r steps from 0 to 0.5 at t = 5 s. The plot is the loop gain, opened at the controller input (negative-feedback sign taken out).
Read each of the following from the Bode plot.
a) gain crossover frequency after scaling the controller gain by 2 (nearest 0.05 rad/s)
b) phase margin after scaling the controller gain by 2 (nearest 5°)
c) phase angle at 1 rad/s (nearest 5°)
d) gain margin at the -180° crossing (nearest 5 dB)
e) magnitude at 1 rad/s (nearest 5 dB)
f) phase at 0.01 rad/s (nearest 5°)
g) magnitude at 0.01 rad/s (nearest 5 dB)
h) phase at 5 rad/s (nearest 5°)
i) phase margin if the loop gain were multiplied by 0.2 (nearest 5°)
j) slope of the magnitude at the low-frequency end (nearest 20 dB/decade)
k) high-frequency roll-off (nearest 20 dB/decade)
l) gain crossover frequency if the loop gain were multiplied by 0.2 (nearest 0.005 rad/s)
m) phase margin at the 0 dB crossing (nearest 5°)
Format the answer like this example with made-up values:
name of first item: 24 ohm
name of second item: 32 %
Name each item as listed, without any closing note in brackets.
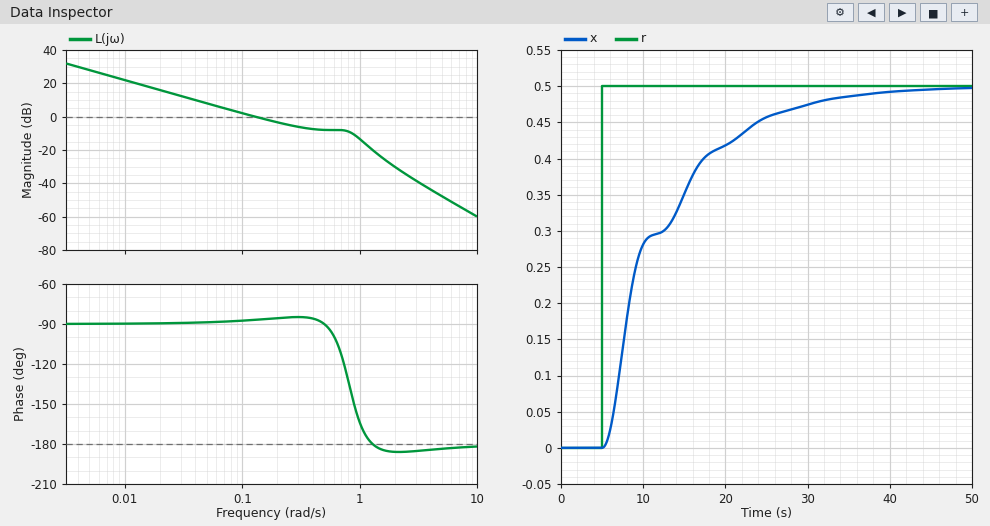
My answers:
gain crossover frequency after scaling the controller gain by 2: 0.30 rad/s
phase margin after scaling the controller gain by 2: 95°
phase angle at 1 rad/s: -165°
gain margin at the -180° crossing: 20 dB
magnitude at 1 rad/s: -15 dB
phase at 0.01 rad/s: -90°
magnitude at 0.01 rad/s: 20 dB
phase at 5 rad/s: -185°
phase margin if the loop gain were multiplied by 0.2: 90°
slope of the magnitude at the low-frequency end: -20 dB/decade
high-frequency roll-off: -40 dB/decade
gain crossover frequency if the loop gain were multiplied by 0.2: 0.025 rad/s
phase margin at the 0 dB crossing: 95°
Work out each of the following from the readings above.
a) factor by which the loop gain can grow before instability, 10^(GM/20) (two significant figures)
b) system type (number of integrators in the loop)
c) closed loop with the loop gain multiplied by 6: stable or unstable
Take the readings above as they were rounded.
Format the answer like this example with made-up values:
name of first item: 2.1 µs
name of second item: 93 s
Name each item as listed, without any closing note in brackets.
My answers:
factor by which the loop gain can grow before instability, 10^(GM/20): 10
system type: 1
closed loop with the loop gain multiplied by 6: stable or unstable: stable
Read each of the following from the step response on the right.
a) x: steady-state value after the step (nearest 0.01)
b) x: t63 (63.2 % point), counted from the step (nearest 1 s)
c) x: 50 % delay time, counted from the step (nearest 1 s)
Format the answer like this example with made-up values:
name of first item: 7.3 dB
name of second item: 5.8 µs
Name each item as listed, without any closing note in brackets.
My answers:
x: steady-state value after the step: 0.50
x: t63 (63.2 % point), counted from the step: 9 s
x: 50 % delay time, counted from the step: 4 s
